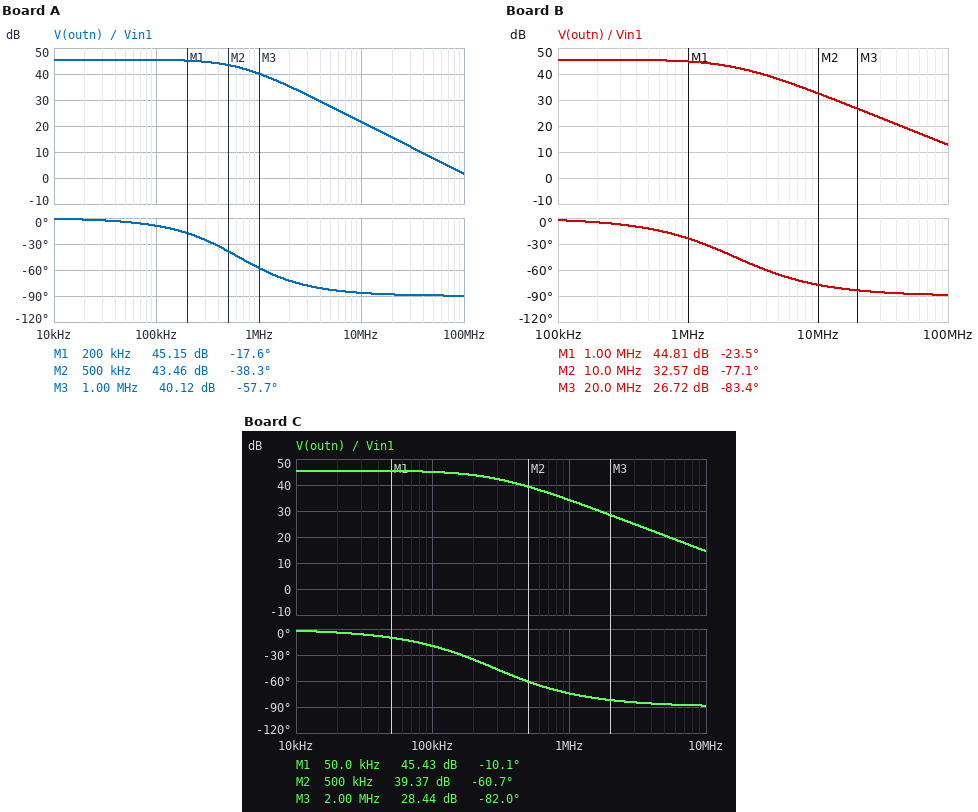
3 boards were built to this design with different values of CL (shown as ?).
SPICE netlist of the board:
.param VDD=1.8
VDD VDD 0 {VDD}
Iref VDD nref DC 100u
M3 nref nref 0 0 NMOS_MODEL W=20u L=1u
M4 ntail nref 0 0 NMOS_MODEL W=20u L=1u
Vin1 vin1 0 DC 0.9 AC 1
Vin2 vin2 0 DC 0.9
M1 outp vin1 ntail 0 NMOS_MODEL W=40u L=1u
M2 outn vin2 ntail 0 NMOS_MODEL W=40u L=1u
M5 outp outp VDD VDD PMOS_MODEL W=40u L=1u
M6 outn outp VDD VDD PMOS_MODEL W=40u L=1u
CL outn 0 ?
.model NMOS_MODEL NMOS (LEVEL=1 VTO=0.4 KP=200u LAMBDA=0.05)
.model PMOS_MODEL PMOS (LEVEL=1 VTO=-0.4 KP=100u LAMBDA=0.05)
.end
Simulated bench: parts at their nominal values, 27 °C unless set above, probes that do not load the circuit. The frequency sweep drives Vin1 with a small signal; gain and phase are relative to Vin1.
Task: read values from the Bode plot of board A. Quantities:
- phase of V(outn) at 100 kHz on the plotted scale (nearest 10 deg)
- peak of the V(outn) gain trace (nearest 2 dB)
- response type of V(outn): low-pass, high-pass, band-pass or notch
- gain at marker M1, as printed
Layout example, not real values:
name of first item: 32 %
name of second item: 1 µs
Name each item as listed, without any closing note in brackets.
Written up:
phase of V(outn) at 100 kHz on the plotted scale: -10 deg
peak of the V(outn) gain trace: 46 dB
response type of V(outn): low-pass, high-pass, band-pass or notch: low-pass
gain at marker M1, as printed: 45.15 dB
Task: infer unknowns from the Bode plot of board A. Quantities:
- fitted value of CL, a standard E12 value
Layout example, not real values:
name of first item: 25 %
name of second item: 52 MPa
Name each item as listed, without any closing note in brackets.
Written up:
fitted value of CL, a standard E12 value: 1.2 pF
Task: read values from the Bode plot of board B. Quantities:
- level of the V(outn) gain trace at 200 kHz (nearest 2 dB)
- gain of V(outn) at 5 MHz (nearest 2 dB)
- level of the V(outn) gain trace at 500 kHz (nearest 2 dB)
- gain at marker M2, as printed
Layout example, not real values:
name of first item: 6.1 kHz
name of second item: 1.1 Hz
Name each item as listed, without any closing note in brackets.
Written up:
level of the V(outn) gain trace at 200 kHz: 46 dB
gain of V(outn) at 5 MHz: 38 dB
level of the V(outn) gain trace at 500 kHz: 46 dB
gain at marker M2, as printed: 32.57 dB
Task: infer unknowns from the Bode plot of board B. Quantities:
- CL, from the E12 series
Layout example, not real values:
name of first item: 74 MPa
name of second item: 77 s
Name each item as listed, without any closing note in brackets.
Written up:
CL, from the E12 series: 330 fF
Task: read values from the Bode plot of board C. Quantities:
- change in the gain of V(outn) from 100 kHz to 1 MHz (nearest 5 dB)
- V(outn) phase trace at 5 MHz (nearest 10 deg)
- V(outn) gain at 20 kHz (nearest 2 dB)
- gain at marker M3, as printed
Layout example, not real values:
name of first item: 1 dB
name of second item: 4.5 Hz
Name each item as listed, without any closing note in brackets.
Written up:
change in the gain of V(outn) from 100 kHz to 1 MHz: -10 dB
V(outn) phase trace at 5 MHz: -90 deg
V(outn) gain at 20 kHz: 46 dB
gain at marker M3, as printed: 28.44 dB
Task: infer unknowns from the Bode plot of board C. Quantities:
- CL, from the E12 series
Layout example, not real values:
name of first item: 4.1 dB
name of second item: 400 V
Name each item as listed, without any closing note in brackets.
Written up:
CL, from the E12 series: 2.7 pF
